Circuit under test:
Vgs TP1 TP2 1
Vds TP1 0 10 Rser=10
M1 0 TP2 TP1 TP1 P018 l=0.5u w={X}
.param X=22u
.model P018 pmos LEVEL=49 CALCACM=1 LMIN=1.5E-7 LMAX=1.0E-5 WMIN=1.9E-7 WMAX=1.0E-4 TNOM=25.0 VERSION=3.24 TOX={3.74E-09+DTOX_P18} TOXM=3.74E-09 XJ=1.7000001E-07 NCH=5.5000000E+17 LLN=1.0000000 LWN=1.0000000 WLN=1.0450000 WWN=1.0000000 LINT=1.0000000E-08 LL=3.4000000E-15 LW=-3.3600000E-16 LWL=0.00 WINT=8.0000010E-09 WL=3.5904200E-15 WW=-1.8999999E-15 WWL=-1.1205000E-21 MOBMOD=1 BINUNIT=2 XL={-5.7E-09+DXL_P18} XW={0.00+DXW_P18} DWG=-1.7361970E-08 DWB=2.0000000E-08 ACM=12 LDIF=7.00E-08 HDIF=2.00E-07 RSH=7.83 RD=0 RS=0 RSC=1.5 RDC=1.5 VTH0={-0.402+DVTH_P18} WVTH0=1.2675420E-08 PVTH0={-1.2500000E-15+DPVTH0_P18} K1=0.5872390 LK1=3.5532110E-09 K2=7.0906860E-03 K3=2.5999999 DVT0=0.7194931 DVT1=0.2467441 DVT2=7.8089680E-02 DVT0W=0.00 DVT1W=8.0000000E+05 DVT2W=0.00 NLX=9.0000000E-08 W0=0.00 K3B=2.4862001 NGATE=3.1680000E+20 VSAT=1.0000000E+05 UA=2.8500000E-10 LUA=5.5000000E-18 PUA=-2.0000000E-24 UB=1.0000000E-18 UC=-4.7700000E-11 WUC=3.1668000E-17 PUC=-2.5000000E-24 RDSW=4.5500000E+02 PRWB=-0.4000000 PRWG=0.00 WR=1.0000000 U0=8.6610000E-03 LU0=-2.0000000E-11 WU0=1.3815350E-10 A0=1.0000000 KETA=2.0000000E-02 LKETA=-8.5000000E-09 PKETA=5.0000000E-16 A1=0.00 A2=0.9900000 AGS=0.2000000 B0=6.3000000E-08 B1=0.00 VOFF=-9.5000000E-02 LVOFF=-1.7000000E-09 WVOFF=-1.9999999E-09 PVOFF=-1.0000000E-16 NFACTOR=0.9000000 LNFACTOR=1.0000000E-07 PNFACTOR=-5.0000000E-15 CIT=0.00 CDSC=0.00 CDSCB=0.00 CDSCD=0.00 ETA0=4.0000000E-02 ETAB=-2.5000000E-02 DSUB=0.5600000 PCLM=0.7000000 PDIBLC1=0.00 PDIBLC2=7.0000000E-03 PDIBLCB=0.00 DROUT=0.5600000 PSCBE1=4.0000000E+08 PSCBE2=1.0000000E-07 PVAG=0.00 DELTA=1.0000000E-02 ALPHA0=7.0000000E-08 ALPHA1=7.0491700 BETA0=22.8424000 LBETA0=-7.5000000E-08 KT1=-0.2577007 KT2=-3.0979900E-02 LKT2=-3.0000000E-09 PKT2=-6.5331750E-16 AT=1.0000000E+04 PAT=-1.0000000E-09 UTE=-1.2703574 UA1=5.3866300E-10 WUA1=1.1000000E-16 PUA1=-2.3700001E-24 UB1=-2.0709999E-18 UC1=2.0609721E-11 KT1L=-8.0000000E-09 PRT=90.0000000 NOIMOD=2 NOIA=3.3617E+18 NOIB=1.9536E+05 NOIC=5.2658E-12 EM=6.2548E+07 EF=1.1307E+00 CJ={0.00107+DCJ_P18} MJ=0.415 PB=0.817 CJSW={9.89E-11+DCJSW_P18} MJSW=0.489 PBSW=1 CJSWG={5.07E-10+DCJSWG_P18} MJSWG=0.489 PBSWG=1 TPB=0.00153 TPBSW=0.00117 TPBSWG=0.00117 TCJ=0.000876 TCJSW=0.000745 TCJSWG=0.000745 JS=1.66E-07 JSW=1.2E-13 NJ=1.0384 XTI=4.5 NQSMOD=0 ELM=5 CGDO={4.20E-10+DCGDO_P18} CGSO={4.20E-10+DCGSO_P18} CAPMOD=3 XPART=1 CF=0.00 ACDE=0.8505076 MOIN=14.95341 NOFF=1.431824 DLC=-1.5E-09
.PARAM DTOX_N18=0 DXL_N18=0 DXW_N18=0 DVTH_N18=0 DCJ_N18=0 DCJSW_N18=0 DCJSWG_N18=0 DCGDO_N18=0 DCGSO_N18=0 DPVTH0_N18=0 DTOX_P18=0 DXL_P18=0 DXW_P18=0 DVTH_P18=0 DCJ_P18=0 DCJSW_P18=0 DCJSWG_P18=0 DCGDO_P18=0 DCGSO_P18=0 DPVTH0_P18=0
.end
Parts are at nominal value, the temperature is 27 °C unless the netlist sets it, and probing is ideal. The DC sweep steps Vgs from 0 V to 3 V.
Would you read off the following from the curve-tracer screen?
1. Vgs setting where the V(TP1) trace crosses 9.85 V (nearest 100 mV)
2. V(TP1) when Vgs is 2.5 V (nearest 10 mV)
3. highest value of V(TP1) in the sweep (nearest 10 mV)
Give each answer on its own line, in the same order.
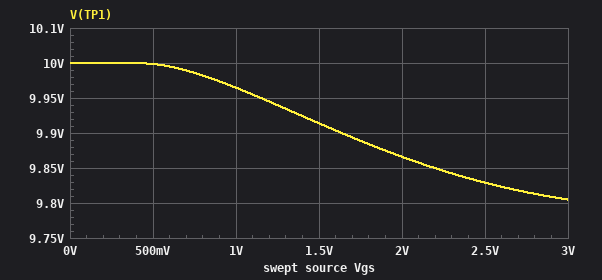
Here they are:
2.2 V
9.83 V
10.00 V
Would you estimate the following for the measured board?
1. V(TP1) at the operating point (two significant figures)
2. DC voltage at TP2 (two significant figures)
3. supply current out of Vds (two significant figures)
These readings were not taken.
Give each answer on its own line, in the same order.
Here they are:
10 V
9.0 V
3.5 mA
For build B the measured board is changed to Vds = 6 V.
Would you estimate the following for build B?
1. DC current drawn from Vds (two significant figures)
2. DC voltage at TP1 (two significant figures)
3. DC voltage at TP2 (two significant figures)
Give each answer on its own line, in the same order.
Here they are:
740 µA
6.0 V
5.0 V
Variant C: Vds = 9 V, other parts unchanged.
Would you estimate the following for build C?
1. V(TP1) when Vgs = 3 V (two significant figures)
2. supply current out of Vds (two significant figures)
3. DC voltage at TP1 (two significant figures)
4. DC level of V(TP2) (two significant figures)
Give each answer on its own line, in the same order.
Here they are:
8.9 V
2.5 mA
9.0 V
8.0 V
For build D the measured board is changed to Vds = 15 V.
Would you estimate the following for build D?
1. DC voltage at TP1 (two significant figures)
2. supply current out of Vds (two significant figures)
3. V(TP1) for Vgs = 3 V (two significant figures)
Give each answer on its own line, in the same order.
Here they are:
15 V
12 mA
14 V
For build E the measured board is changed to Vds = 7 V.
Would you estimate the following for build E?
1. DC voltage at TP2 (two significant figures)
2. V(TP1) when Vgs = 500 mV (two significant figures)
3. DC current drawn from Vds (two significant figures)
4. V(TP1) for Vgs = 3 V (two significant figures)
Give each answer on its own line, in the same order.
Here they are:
6.0 V
7.0 V
1.1 mA
6.9 V
